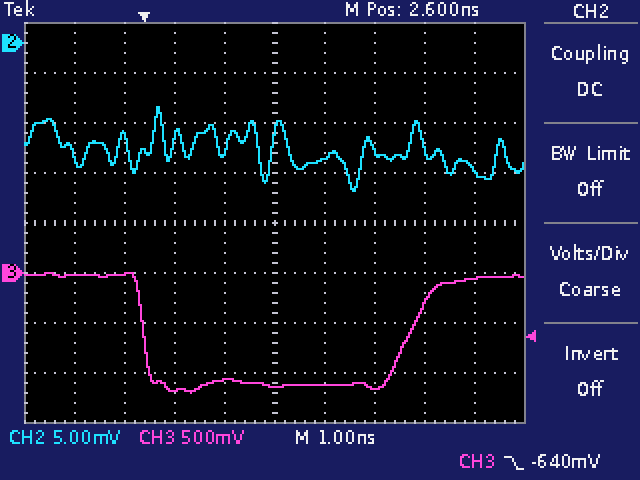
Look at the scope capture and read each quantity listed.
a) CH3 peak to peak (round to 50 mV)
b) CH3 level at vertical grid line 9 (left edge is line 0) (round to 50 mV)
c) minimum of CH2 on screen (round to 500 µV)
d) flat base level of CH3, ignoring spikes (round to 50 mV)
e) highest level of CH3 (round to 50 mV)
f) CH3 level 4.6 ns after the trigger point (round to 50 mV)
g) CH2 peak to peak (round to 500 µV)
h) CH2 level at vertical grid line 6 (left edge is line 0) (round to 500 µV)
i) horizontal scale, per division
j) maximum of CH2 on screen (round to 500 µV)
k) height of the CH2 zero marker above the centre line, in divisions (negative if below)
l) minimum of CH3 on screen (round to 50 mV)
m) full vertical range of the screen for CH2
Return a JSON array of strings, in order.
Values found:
["1.20 V", "-50 mV", "-15.0 mV", "-1.10 V", "0 mV", "-1.15 V", "8.5 mV", "-11.5 mV", "1 ns", "-6.5 mV", "+3.6 div", "-1.20 V", "40 mV"]
